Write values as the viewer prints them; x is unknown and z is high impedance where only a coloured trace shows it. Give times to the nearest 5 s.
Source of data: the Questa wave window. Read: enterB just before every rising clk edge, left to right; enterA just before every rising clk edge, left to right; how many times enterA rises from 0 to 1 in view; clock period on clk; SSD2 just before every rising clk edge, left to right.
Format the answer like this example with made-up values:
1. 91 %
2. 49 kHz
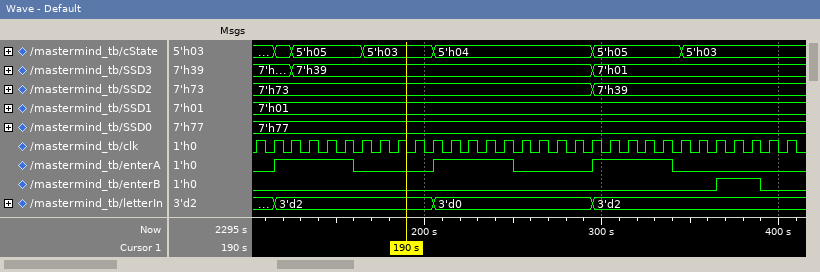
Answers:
1. 0 0 0 0 0 0 0 0 0 0 0 0 0 0 0 0 0 0 0 0 0 0 0 0 0 0 0 1 1 0 0
2. 0 0 1 1 1 1 0 0 0 0 0 1 1 1 1 0 0 0 0 0 1 1 1 1 0 0 0 0 0 0 0
3. 3
4. 10 s
5. 7'h73, 7'h73, 7'h73, 7'h73, 7'h73, 7'h73, 7'h73, 7'h73, 7'h73, 7'h73, 7'h73, 7'h73, 7'h73, 7'h73, 7'h73, 7'h73, 7'h73, 7'h73, 7'h73, 7'h73, 7'h39, 7'h39, 7'h39, 7'h39, 7'h39, 7'h39, 7'h39, 7'h39, 7'h39, 7'h39, 7'h39
